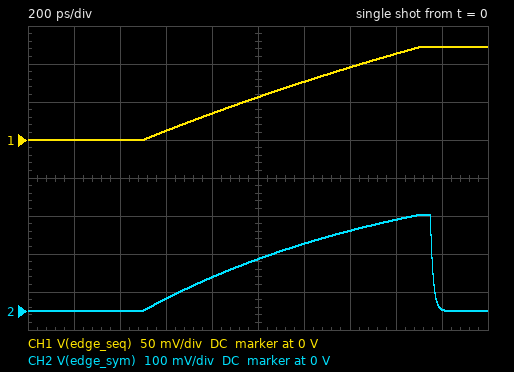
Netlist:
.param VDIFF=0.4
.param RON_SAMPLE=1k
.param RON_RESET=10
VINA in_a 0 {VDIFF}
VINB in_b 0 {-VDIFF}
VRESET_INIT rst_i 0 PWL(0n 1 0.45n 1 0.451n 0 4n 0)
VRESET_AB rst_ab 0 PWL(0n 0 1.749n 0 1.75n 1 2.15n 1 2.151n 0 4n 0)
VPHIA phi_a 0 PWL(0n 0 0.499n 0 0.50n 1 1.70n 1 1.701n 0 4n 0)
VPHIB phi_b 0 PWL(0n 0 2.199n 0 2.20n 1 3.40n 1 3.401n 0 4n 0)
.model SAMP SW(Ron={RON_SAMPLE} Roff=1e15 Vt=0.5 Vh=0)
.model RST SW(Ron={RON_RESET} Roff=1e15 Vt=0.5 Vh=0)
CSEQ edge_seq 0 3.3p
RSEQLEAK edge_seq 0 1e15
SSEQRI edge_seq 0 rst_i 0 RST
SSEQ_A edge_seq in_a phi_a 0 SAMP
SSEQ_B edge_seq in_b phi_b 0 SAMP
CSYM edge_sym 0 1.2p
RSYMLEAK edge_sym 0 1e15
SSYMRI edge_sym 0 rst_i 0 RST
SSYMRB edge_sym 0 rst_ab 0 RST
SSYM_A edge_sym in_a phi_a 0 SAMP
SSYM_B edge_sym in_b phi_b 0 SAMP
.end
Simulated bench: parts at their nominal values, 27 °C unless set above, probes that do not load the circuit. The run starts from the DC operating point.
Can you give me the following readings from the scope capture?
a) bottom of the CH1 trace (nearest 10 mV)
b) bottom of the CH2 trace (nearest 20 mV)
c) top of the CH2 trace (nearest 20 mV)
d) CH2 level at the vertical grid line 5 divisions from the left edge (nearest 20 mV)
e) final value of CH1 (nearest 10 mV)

0 V
0 V
260 mV
140 mV
120 mV
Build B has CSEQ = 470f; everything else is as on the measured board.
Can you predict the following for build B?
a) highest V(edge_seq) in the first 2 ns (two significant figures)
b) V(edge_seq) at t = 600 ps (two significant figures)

370 mV
77 mV
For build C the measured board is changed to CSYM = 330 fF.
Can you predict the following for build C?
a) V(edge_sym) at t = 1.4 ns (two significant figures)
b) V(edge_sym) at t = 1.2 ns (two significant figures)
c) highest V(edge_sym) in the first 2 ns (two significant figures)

370 mV
350 mV
390 mV
